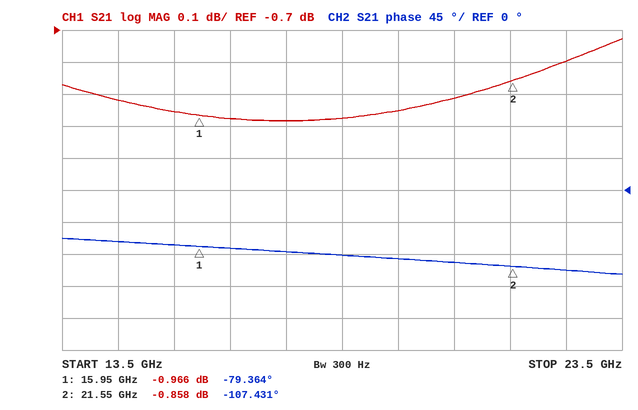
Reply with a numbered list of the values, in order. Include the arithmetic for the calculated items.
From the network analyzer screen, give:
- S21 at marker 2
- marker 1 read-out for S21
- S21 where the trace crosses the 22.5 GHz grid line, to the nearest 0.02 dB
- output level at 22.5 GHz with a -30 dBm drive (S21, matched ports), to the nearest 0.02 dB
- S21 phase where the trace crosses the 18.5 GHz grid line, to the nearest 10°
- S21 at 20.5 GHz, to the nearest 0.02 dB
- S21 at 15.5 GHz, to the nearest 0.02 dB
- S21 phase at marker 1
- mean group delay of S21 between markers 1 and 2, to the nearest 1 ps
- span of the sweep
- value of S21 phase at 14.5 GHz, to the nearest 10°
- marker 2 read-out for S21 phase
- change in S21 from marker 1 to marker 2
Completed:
1. -0.858 dB
2. -0.966 dB
3. -0.80 dB
4. -30 dBm + (-0.80 dB) = -30.80 dBm
5. -90°
6. -0.92 dB
7. -0.96 dB
8. -79.364°
9. −(-107.431° − (-79.364°))/(360° × 5.6 GHz) ≈ 14 ps
10. 10 GHz
11. -70°
12. -107.431°
13. -0.858 − (-0.966) = 0.108 dB
